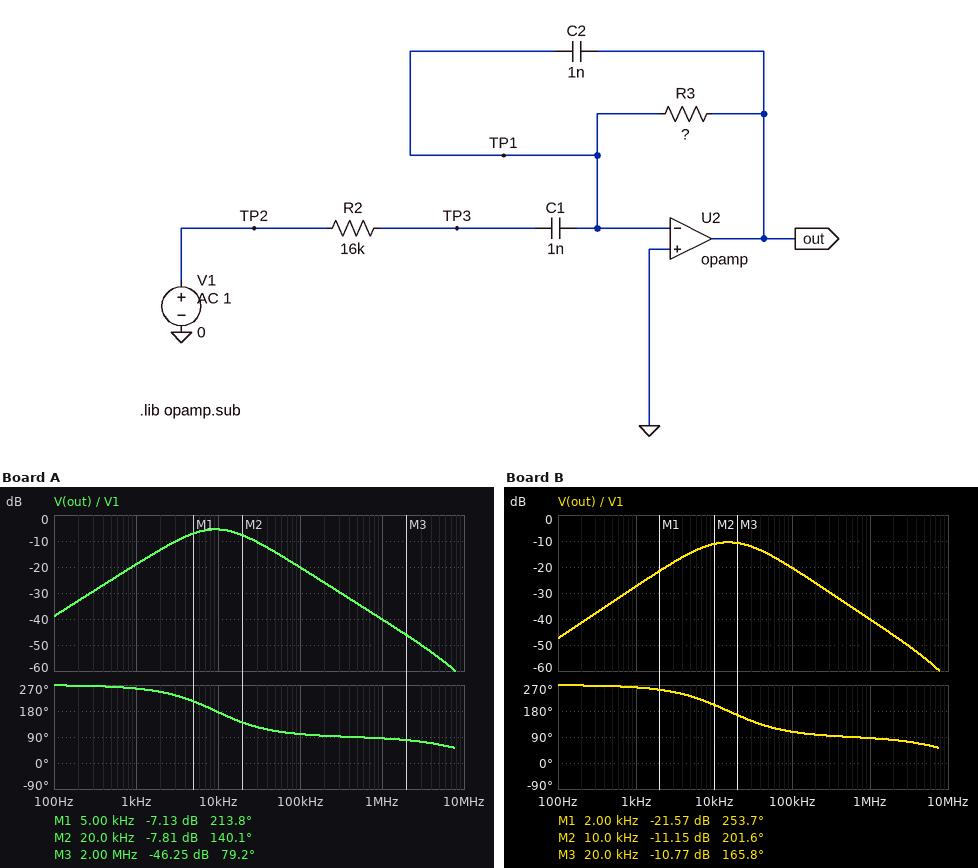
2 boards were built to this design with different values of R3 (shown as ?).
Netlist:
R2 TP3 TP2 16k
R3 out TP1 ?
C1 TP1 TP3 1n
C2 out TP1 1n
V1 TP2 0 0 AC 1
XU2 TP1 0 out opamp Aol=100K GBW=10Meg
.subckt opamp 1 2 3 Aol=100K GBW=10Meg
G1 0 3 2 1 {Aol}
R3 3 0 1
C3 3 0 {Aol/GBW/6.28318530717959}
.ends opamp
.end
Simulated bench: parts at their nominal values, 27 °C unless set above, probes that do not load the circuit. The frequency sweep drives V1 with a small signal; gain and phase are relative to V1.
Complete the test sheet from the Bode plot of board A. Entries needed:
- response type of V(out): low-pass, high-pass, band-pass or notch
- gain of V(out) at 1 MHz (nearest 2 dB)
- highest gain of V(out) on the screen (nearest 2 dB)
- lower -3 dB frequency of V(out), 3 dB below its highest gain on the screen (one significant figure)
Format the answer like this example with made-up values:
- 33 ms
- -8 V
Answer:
- band-pass
- -40 dB
- -6 dB
- 4 kHz
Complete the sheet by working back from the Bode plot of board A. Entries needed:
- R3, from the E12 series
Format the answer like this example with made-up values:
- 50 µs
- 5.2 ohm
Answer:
- 18 kΩ
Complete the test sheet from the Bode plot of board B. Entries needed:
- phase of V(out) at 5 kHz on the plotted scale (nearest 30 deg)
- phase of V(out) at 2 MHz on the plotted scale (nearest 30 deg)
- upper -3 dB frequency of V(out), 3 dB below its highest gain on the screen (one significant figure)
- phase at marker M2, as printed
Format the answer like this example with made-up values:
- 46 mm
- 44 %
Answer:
- 240 deg
- 90 deg
- 40 kHz
- 201.6 deg
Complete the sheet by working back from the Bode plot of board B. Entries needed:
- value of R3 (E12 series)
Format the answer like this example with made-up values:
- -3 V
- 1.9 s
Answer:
- 6.8 kΩ
